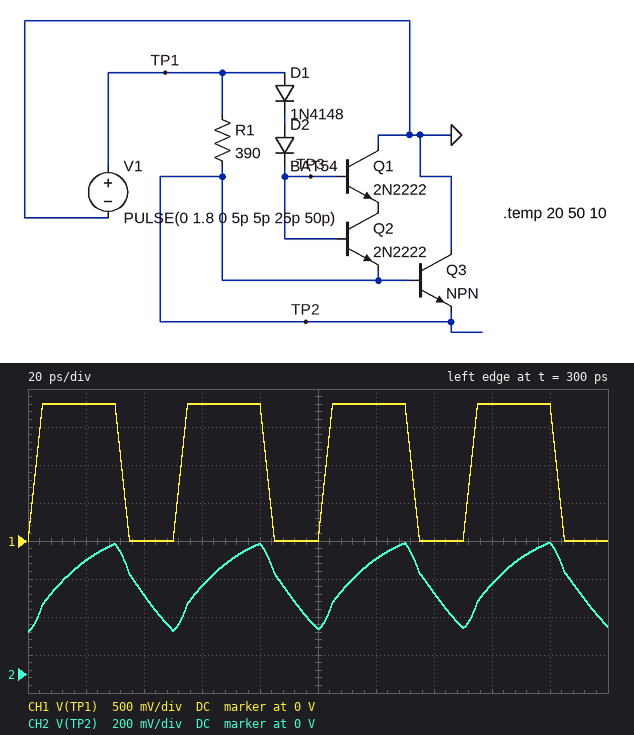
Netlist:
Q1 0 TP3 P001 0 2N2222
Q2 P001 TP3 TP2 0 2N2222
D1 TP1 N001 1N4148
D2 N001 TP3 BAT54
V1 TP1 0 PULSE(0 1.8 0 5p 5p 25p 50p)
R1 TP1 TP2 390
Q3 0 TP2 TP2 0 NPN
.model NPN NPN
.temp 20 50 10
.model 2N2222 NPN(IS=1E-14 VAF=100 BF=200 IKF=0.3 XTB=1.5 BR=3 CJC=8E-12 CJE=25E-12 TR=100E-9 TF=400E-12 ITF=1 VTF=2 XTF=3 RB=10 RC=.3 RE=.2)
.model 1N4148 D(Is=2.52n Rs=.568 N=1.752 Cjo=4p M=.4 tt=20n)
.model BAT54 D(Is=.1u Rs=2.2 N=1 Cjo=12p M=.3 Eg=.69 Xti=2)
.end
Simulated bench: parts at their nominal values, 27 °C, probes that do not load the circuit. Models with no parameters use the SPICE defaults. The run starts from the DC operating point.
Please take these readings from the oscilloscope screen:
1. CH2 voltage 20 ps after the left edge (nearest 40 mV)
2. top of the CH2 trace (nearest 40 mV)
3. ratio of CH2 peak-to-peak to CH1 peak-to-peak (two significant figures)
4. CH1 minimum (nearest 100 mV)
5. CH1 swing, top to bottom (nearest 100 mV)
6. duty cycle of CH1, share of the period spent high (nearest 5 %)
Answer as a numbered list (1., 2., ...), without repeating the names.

1. 600 mV
2. 680 mV
3. 0.26
4. 0 V
5. 1.8 V
6. 60 %
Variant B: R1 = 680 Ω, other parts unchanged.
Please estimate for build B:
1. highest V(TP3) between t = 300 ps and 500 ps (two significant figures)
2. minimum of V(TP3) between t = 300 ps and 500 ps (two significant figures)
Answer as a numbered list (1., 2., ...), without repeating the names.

1. 940 mV
2. -320 mV
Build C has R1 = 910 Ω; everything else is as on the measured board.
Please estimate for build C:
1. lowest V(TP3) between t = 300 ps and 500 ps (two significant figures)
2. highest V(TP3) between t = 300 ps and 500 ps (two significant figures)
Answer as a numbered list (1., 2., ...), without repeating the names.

1. -320 mV
2. 930 mV
